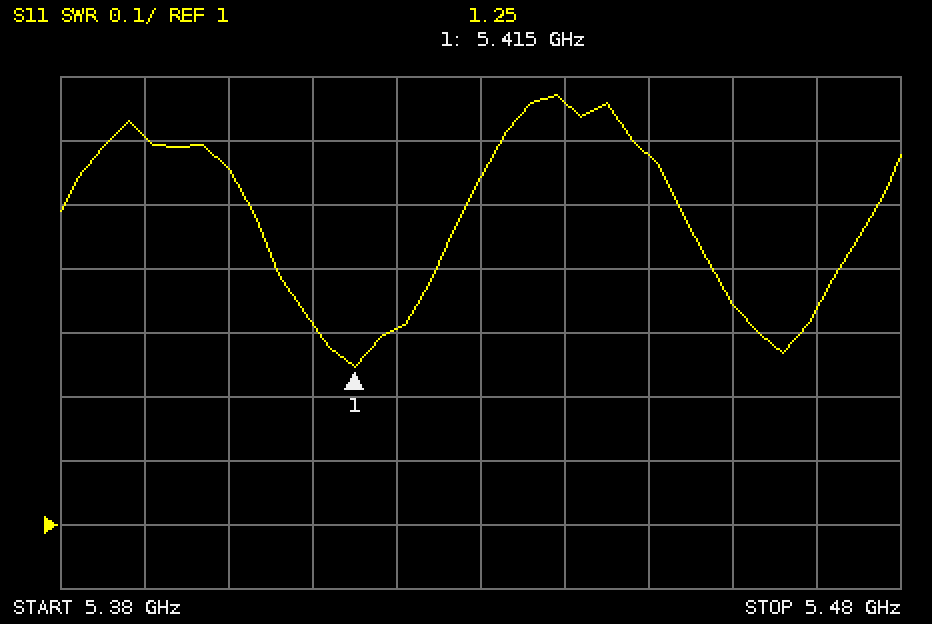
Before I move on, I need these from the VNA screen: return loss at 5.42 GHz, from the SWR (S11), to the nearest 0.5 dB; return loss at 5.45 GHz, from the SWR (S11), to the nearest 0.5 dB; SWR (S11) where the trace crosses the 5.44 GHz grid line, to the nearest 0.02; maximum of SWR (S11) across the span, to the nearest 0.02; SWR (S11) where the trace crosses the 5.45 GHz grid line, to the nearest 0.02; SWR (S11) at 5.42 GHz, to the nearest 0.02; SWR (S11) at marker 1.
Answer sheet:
17.5 dB
13.0 dB
1.66
1.68
1.58
1.30
1.25
